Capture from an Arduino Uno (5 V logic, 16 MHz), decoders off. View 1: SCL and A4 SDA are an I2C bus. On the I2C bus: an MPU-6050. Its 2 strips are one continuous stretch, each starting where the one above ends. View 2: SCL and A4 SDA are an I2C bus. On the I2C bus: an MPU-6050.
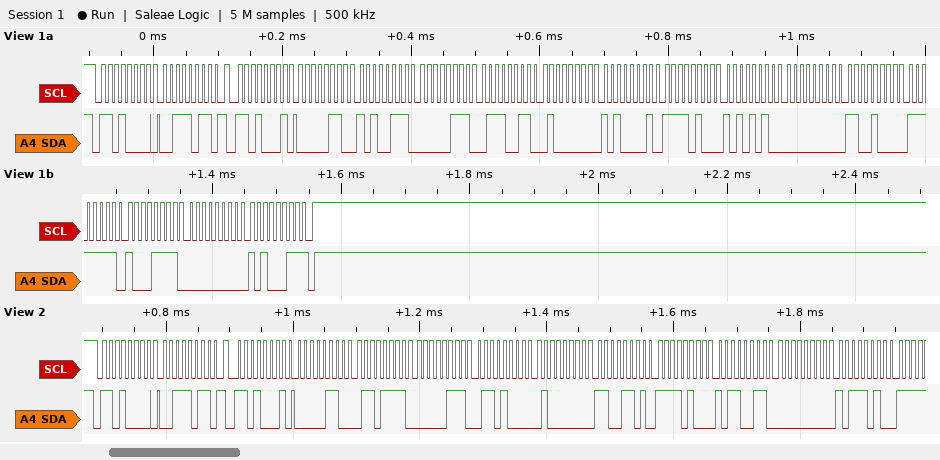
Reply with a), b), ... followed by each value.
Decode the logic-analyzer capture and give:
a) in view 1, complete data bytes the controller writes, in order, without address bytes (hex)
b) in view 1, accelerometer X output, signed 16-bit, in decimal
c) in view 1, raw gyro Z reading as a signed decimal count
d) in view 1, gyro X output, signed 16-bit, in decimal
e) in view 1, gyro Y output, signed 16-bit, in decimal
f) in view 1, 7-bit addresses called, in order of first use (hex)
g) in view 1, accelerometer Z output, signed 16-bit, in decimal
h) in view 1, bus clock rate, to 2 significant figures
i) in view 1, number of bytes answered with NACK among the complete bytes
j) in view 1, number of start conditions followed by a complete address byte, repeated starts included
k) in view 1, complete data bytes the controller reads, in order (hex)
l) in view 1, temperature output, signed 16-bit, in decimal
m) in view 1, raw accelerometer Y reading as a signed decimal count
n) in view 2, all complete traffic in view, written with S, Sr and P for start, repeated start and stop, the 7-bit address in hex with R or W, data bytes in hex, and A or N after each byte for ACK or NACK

a) 3B
b) 1703
c) 163
d) 200
e) -113
f) 0x68
g) 16545
h) 100 kHz
i) 1
j) 2
k) 06 A7 07 73 40 A1 F4 AA 00 C8 FF 8F 00 A3
l) -2902
m) 1907
n) S 68W A 3B A Sr 68R A 06 A 6F A 07 A 68 A 40 A CD A F4 A B3 A 00 A BA A
